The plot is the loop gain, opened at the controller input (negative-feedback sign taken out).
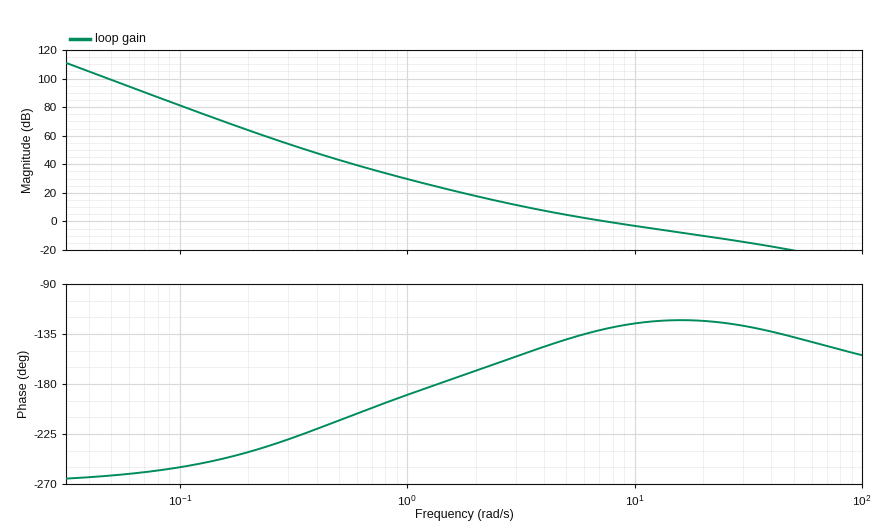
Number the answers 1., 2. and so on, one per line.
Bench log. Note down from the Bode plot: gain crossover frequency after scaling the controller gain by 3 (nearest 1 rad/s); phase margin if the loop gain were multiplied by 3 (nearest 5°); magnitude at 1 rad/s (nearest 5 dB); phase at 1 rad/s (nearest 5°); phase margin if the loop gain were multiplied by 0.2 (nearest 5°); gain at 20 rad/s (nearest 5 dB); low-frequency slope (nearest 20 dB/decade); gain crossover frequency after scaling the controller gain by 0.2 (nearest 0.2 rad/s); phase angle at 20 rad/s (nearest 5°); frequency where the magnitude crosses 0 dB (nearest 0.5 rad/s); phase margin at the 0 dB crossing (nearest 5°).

1. 19 rad/s
2. 55°
3. 30 dB
4. -190°
5. 20°
6. -10 dB
7. -60 dB/decade
8. 2.6 rad/s
9. -125°
10. 7.5 rad/s
11. 50°
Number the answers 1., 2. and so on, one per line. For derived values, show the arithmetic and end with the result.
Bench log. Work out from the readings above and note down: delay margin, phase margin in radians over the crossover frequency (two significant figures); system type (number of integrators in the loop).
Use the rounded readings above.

1. 50 × π / 180 / 7.5 = 0.12 s
2. 3
